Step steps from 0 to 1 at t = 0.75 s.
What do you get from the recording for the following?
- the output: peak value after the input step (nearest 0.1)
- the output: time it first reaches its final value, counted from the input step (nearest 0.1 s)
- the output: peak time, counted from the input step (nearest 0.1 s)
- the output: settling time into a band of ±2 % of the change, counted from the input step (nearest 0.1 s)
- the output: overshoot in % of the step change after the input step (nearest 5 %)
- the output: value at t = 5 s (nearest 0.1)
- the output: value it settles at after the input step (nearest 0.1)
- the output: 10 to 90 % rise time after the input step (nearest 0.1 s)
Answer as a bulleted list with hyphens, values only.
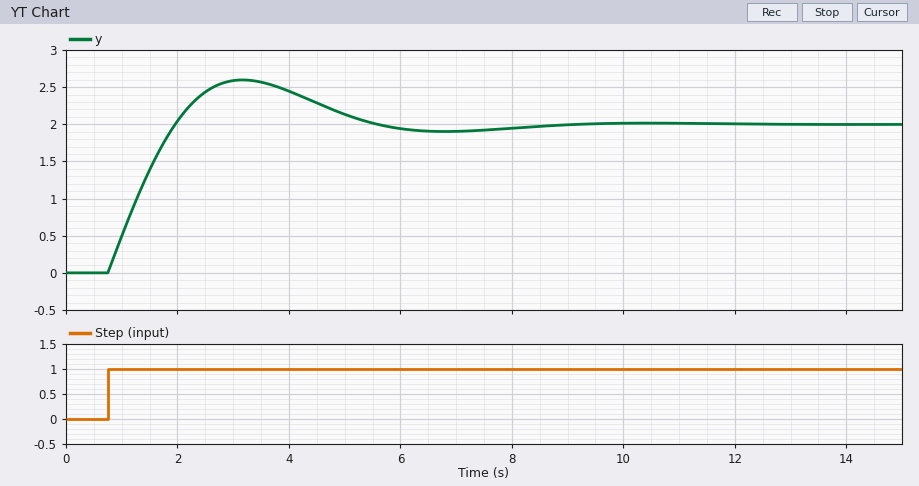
- 2.6
- 1.2 s
- 2.4 s
- 7.5 s
- 30 %
- 2.1
- 2.0
- 0.9 s
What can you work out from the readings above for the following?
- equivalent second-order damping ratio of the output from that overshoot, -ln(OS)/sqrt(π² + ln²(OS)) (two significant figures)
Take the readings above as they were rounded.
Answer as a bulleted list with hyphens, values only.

- 0.36
